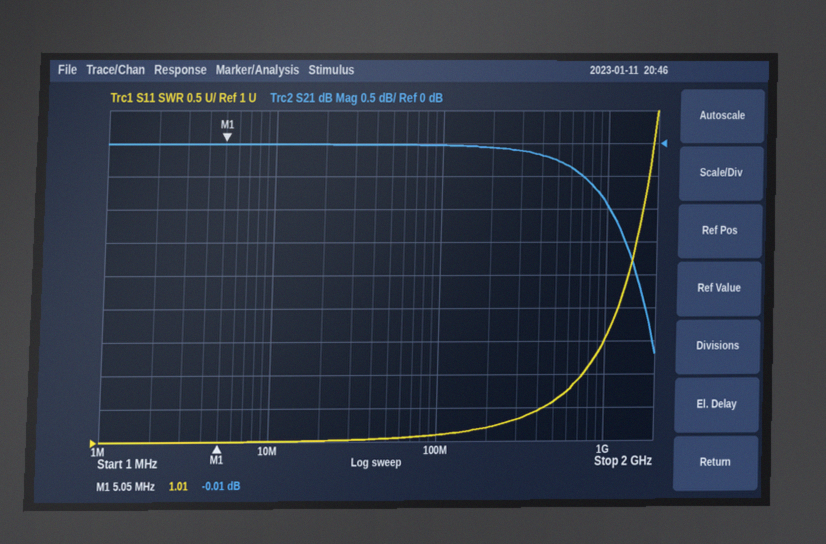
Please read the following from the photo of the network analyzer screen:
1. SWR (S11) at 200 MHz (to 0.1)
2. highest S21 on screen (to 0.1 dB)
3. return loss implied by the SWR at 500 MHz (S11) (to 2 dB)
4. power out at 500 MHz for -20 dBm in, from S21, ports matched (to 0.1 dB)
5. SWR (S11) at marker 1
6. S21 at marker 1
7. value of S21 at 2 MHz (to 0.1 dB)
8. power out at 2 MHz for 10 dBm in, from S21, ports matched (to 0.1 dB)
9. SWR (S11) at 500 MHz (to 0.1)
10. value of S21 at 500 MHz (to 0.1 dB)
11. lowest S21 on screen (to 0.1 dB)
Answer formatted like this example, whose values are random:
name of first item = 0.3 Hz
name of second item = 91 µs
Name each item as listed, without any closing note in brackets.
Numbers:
SWR (S11) at 200 MHz = 1.2
highest S21 on screen = 0.0 dB
return loss implied by the SWR at 500 MHz (S11) = 12 dB
power out at 500 MHz for -20 dBm in, from S21, ports matched = -20.3 dBm
SWR (S11) at marker 1 = 1.01
S21 at marker 1 = -0.01 dB
value of S21 at 2 MHz = 0.0 dB
power out at 2 MHz for 10 dBm in, from S21, ports matched = 10.0 dBm
SWR (S11) at 500 MHz = 1.6
value of S21 at 500 MHz = -0.3 dB
lowest S21 on screen = -3.2 dB
